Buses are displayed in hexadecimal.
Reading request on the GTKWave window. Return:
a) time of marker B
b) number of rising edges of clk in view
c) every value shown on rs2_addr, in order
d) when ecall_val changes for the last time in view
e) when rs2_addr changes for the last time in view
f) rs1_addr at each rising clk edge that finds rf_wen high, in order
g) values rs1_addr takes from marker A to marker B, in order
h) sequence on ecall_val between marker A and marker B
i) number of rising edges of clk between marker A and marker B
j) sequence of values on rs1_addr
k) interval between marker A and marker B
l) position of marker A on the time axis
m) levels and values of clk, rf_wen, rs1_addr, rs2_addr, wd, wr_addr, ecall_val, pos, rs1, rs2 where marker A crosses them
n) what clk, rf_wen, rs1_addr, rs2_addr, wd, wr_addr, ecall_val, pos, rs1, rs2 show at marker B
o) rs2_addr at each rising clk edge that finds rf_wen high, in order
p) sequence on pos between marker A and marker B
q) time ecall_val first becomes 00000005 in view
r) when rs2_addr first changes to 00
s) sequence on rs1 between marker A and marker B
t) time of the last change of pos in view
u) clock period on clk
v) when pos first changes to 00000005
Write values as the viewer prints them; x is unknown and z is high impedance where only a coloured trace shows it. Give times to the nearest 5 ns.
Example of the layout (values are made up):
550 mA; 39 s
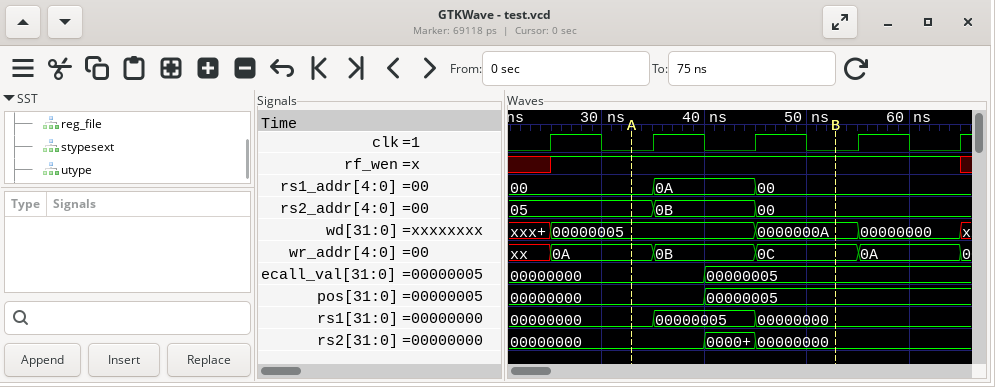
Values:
55 ns; 5; 05, 0B, 00; 40 ns; 45 ns; 00, 0A, 00, 00; 00, 0A, 00; 00000000, 00000005; 2; 00, 0A, 00; 20 ns; 35 ns; clk=0, rf_wen=1, rs1_addr=00, rs2_addr=05, wd=00000005, wr_addr=0A, ecall_val=00000000, pos=00000000, rs1=00000000, rs2=00000000; clk=0, rf_wen=1, rs1_addr=00, rs2_addr=00, wd=0000000A, wr_addr=0C, ecall_val=00000005, pos=00000005, rs1=00000000, rs2=00000000; 05, 0B, 00, 00; 00000000, 00000005; 40 ns; 45 ns; 00000000, 00000005, 00000000; 40 ns; 10 ns; 40 ns
